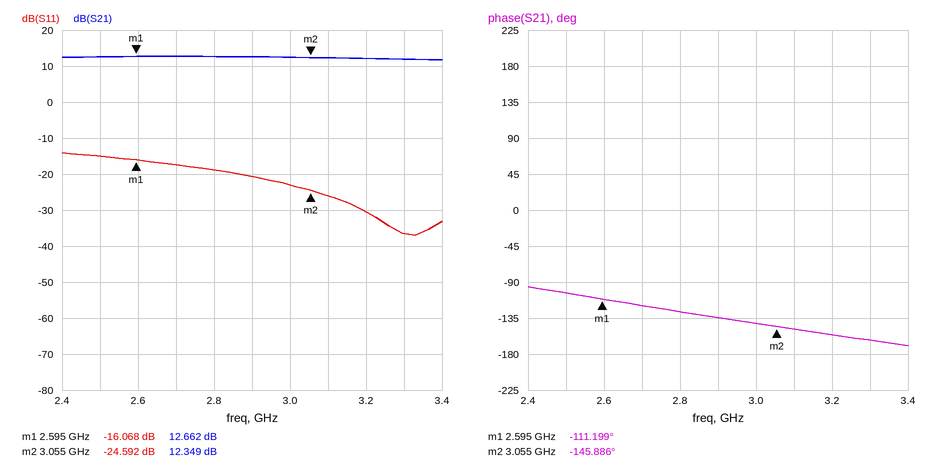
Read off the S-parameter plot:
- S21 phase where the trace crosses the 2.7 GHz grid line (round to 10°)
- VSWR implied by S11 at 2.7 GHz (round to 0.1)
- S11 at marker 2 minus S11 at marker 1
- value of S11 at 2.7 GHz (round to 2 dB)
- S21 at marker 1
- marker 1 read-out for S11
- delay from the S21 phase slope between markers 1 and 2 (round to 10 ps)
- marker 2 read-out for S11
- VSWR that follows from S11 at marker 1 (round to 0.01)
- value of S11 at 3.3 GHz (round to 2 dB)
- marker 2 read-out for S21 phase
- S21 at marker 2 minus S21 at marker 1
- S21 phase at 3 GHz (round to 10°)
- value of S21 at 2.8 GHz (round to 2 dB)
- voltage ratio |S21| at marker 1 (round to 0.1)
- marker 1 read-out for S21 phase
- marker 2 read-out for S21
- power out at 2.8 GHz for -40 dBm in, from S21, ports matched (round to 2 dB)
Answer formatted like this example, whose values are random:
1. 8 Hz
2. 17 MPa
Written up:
1. -120°
2. 1.3
3. -8.524 dB
4. -18 dB
5. 12.662 dB
6. -16.068 dB
7. 210 ps
8. -24.592 dB
9. 1.37
10. -36 dB
11. -145.886°
12. -0.313 dB
13. -140°
14. 12 dB
15. 4.3
16. -111.199°
17. 12.349 dB
18. -28 dBm
